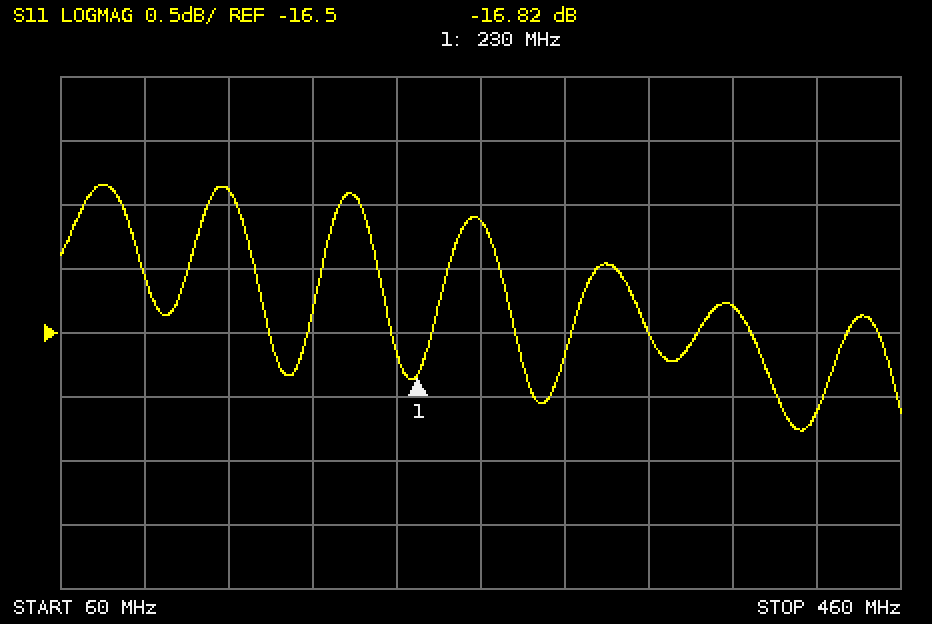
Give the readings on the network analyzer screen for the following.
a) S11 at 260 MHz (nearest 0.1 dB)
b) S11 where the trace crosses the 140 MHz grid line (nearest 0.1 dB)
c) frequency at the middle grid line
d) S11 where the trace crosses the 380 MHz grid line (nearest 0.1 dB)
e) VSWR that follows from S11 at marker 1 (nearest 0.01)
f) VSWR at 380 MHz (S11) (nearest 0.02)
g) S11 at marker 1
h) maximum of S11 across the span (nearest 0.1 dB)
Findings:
-15.6 dB
-15.4 dB
260 MHz
-16.3 dB
1.34
1.36
-16.82 dB
-15.3 dB
